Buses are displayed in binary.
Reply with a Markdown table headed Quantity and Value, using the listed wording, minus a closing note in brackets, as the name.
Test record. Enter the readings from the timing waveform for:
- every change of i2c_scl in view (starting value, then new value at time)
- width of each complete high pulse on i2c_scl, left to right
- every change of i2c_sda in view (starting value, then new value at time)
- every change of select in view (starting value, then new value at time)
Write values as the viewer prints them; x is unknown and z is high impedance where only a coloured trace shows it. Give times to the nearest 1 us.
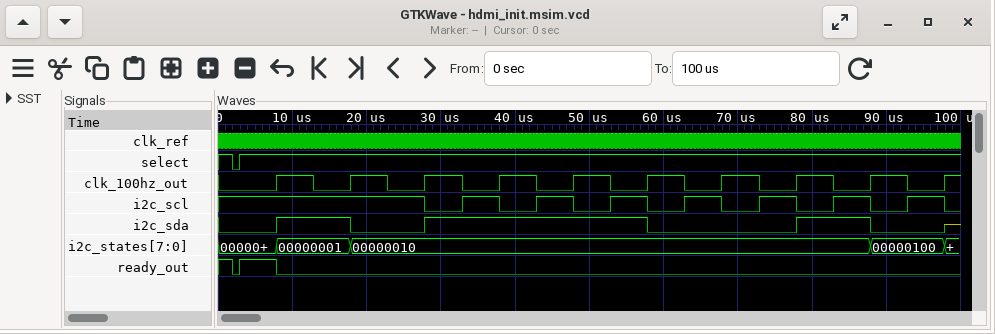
| Quantity | Value |
|---|---|
| every change of i2c_scl in view | 1, 0 at 28 us, 1 at 33 us, 0 at 38 us, 1 at 43 us, 0 at 48 us, 1 at 53 us, 0 at 58 us, 1 at 63 us, 0 at 68 us, 1 at 73 us, 0 at 78 us, 1 at 83 us, 0 at 88 us, 1 at 93 us, 0 at 98 us |
| width of each complete high pulse on i2c_scl, left to right | 5 us, 5 us, 5 us, 5 us, 5 us, 5 us, 5 us |
| every change of i2c_sda in view | 0, 1 at 8 us, 0 at 18 us, 1 at 28 us, 0 at 58 us, 1 at 78 us, 0 at 88 us, z at 98 us |
| every change of select in view | 1, 0 at 2 us, 1 at 3 us |
